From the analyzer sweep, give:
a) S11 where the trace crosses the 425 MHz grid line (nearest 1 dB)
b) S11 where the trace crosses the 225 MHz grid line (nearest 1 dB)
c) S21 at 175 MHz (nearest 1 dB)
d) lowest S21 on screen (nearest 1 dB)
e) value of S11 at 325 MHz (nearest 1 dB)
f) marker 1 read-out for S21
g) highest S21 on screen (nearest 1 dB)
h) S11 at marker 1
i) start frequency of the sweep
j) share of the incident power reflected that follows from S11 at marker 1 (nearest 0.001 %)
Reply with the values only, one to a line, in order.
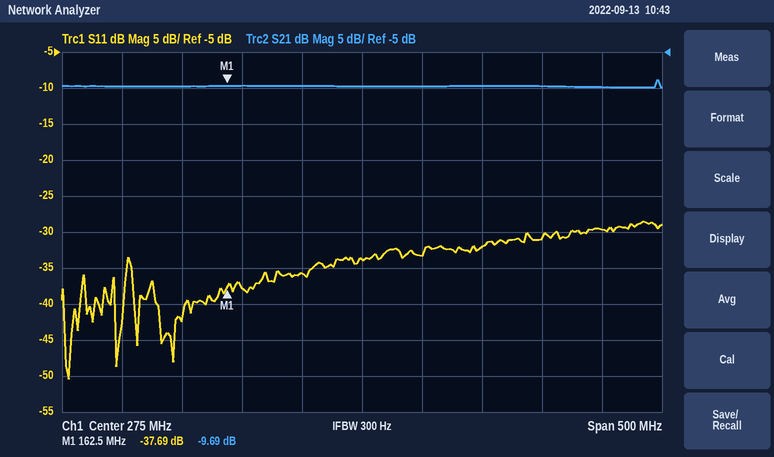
-31 dB
-36 dB
-10 dB
-10 dB
-33 dB
-9.69 dB
-9 dB
-37.69 dB
25 MHz
0.017 %
